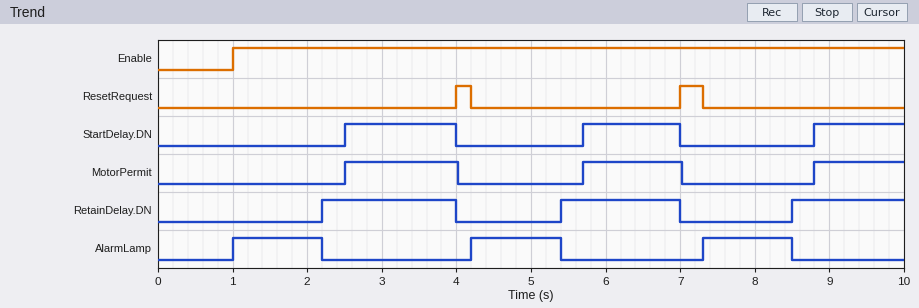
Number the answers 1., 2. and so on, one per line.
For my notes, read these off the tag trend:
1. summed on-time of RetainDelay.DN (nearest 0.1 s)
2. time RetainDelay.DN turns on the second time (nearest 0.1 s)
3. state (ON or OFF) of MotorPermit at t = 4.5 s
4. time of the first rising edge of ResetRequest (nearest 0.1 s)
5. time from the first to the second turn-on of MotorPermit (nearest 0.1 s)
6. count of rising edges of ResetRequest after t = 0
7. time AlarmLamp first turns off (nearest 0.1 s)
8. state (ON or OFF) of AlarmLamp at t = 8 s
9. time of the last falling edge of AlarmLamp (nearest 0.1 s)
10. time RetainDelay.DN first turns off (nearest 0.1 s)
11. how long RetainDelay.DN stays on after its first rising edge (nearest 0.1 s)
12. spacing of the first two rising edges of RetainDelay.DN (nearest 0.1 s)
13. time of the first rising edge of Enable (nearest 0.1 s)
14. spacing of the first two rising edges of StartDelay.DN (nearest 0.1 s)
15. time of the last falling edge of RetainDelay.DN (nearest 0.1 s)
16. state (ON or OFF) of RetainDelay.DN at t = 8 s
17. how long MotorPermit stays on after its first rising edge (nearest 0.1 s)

1. 4.9 s
2. 5.4 s
3. OFF
4. 4.0 s
5. 3.2 s
6. 2
7. 2.2 s
8. ON
9. 8.5 s
10. 4.0 s
11. 1.8 s
12. 3.2 s
13. 1.0 s
14. 3.2 s
15. 7.0 s
16. OFF
17. 1.5 s
